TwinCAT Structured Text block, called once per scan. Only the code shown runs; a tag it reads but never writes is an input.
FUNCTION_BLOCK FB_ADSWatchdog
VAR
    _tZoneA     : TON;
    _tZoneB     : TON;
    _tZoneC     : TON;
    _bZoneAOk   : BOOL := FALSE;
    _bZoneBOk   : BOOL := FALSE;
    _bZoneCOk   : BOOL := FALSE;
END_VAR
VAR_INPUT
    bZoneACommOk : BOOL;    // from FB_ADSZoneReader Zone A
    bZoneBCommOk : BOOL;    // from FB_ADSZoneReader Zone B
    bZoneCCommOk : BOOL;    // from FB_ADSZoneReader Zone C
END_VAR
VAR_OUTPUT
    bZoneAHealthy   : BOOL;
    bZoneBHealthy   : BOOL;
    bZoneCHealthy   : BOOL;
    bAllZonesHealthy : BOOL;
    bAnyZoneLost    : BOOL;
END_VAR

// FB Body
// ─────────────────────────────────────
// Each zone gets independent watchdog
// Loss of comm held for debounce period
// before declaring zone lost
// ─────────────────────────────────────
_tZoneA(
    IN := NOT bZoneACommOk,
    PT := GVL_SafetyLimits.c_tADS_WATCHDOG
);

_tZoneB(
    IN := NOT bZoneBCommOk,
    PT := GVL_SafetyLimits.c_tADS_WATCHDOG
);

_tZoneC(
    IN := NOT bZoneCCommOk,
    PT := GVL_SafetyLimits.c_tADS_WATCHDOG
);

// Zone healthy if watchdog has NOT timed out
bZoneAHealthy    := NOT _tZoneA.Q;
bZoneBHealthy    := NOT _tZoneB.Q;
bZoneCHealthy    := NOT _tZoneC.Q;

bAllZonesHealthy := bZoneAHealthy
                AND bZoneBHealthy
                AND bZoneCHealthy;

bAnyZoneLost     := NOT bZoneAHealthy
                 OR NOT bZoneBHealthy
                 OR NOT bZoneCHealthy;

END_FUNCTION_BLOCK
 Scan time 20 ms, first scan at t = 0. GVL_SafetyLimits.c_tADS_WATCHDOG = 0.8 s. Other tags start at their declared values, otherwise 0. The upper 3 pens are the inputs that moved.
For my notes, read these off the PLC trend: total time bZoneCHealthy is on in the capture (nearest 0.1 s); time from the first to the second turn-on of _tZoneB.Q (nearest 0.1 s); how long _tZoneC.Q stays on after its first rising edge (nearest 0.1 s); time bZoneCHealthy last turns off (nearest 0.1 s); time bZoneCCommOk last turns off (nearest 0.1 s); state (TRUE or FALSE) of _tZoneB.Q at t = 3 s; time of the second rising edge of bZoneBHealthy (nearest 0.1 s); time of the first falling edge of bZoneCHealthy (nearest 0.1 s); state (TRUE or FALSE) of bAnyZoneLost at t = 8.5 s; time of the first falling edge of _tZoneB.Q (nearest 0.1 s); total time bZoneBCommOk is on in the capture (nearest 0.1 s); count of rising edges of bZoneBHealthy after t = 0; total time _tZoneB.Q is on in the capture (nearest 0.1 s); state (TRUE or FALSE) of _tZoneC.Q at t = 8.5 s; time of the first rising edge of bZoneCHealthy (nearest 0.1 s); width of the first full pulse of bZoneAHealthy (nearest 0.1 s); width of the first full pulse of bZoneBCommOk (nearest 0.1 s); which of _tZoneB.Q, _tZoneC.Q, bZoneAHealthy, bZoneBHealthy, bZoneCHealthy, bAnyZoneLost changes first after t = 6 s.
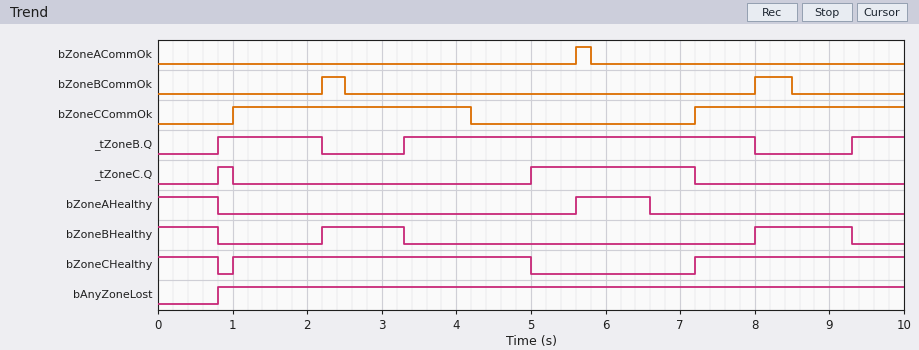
7.6 s
2.5 s
0.2 s
5.0 s
4.2 s
FALSE
8.0 s
0.8 s
TRUE
2.2 s
0.8 s
2
6.8 s
FALSE
1.0 s
1.0 s
0.3 s
bZoneAHealthy
